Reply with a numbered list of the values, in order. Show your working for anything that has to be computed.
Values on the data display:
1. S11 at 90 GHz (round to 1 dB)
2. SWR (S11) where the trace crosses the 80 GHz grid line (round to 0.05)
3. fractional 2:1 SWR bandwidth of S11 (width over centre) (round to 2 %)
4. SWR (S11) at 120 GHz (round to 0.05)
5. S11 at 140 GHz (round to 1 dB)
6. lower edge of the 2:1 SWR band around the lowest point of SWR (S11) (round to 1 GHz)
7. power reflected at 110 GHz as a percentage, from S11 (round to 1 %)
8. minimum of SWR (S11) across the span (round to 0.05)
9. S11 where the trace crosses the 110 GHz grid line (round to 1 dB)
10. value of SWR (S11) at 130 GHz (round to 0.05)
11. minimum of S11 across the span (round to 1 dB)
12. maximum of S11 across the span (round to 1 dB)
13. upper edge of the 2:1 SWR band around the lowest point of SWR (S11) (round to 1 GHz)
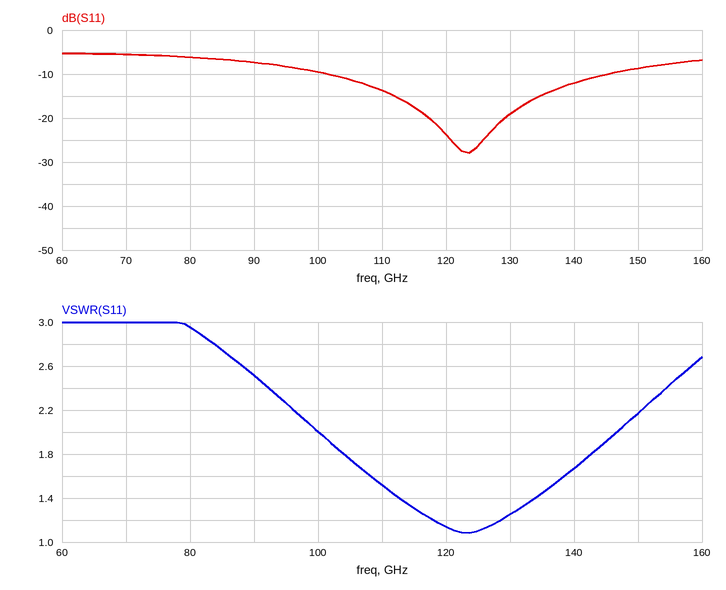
1. -7 dB
2. 2.95
3. 47 GHz / 123.5 GHz ≈ 38 %
4. 1.15
5. -12 dB
6. 100 GHz
7. 10^(-14/10) ≈ 4 %
8. 1.10
9. -14 dB
10. 1.25
11. -28 dB
12. -5 dB
13. 147 GHz
